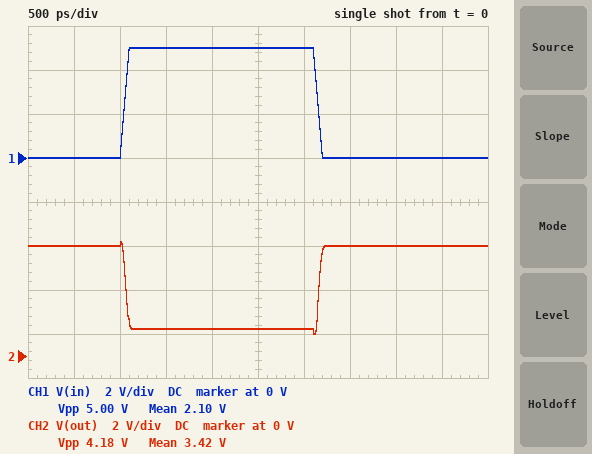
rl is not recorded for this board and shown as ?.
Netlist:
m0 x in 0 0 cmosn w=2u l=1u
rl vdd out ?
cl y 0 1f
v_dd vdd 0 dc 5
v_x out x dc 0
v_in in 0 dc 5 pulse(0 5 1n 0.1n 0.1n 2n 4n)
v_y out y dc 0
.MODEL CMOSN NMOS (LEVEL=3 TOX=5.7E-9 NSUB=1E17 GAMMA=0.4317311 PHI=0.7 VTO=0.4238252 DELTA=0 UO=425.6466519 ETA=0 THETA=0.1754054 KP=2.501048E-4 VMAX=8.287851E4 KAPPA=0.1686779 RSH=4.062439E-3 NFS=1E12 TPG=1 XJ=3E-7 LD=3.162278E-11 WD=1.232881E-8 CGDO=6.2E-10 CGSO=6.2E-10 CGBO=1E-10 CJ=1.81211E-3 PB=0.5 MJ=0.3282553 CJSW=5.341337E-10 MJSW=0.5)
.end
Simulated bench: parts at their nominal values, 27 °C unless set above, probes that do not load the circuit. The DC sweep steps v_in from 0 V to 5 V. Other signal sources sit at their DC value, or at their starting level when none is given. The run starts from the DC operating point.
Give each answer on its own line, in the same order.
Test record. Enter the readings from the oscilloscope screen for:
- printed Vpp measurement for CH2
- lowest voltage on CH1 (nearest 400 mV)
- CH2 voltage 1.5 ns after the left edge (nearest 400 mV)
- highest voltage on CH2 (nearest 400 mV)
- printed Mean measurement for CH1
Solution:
4.18 V
0 V
1.2 V
5.2 V
2.10 V
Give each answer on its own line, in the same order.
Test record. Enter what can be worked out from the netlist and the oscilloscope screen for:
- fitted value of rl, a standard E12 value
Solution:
3.9 kΩ
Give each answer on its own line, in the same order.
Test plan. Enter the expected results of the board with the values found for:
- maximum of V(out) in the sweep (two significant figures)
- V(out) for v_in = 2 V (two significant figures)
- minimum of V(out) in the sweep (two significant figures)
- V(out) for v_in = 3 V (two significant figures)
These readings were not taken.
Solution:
5.0 V
3.8 V
1.2 V
2.6 V
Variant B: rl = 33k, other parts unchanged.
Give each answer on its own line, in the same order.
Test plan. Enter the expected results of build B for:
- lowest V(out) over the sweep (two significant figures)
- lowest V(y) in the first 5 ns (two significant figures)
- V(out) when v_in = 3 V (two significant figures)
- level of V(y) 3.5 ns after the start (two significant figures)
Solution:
120 mV
-620 mV
180 mV
4.9 V
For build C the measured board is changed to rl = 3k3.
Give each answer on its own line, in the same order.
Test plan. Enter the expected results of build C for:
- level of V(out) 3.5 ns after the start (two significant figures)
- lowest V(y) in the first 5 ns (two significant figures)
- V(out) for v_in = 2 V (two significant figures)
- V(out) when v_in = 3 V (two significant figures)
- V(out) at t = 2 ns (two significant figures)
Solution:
5.0 V
1.3 V
4.0 V
3.0 V
1.5 V
